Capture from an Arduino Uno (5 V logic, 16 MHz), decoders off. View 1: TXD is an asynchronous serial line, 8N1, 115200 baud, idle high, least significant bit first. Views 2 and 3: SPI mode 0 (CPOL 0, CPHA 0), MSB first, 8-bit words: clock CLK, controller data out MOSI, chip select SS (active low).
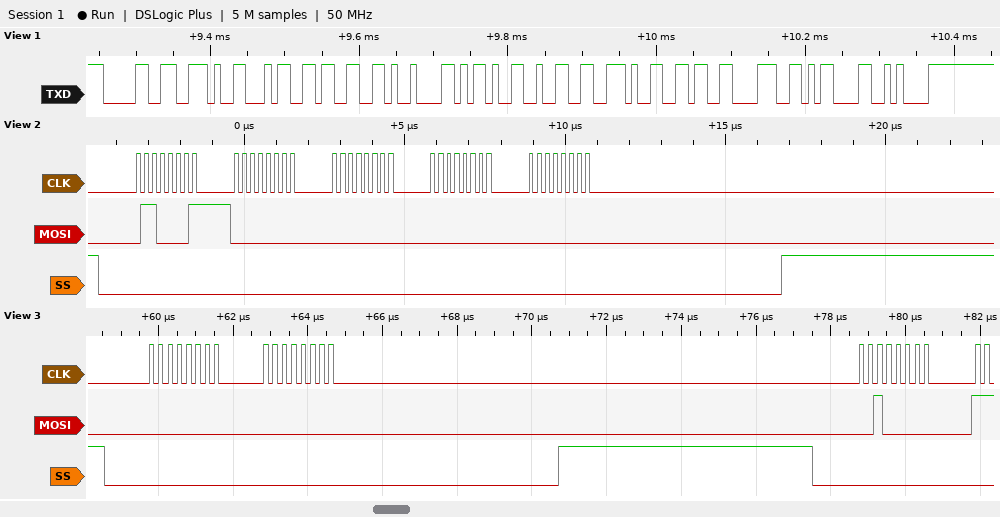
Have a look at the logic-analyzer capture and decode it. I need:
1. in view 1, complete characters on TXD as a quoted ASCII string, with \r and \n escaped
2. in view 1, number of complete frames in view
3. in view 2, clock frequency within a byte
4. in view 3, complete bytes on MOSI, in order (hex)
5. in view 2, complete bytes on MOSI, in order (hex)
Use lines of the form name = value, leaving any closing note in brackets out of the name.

in view 1, complete characters on TXD as a quoted ASCII string, with \r and \n escaped = "0.43\t-2.68\r\n"
in view 1, number of complete frames in view = 12
in view 2, clock frequency within a byte = 4 MHz
in view 3, complete bytes on MOSI, in order = 00 00 20
in view 2, complete bytes on MOSI, in order = 61 00 00 00 00
